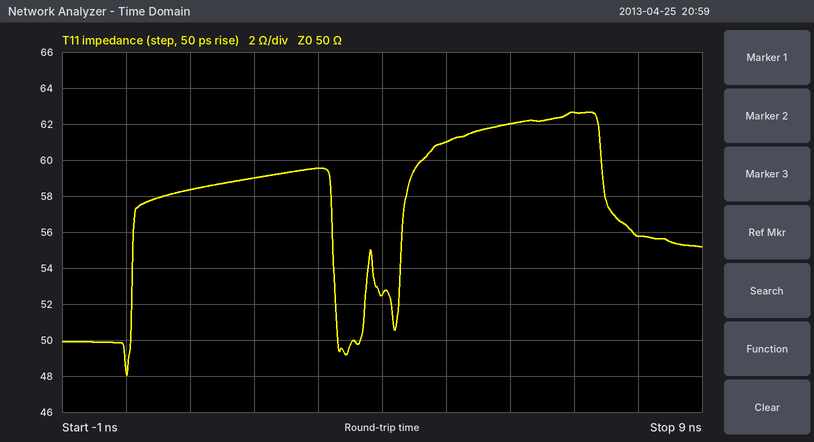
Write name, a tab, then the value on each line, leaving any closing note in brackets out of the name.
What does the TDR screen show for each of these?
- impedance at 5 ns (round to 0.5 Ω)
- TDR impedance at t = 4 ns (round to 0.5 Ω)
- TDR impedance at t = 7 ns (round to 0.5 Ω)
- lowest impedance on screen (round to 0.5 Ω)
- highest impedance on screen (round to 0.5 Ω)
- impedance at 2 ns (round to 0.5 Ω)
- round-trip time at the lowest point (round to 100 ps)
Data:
impedance at 5 ns	61.0 Ω
TDR impedance at t = 4 ns	52.5 Ω
TDR impedance at t = 7 ns	62.5 Ω
lowest impedance on screen	48.0 Ω
highest impedance on screen	62.5 Ω
impedance at 2 ns	59.0 Ω
round-trip time at the lowest point	0.0 ns
